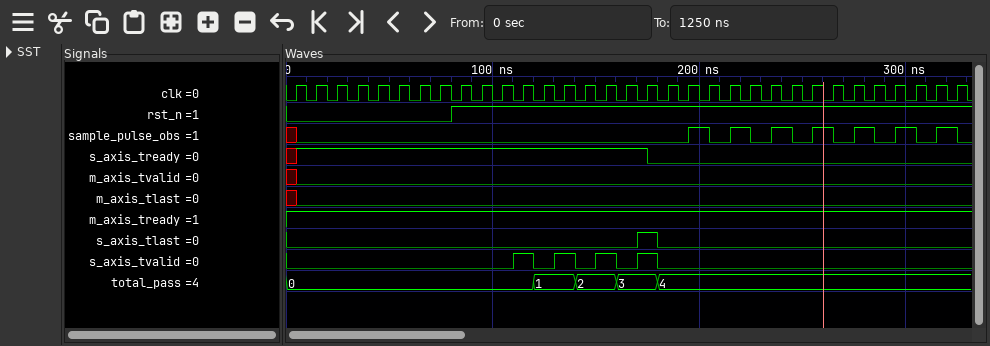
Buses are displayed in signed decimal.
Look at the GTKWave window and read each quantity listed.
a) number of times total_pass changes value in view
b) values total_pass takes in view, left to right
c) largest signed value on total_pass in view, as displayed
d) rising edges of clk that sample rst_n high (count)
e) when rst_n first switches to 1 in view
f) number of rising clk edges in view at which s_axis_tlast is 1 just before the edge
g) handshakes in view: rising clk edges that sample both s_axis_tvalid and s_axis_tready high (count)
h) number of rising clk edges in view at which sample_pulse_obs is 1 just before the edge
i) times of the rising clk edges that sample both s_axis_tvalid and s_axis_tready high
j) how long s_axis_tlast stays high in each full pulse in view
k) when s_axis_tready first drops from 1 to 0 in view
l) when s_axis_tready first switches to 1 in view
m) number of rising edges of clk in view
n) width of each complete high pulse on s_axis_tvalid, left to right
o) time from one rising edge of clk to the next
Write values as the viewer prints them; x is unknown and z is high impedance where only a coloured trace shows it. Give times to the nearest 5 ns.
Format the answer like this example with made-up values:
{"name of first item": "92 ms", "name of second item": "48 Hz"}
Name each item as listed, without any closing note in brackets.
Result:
{"number of times total_pass changes value in view": "4", "values total_pass takes in view, left to right": "0, 1, 2, 3, 4", "largest signed value on total_pass in view, as displayed": "4", "rising edges of clk that sample rst_n high": "25", "when rst_n first switches to 1 in view": "80 ns", "number of rising clk edges in view at which s_axis_tlast is 1 just before the edge": "1", "handshakes in view: rising clk edges that sample both s_axis_tvalid and s_axis_tready high": "4", "number of rising clk edges in view at which sample_pulse_obs is 1 just before the edge": "7", "times of the rising clk edges that sample both s_axis_tvalid and s_axis_tready high": "115 ns, 135 ns, 155 ns, 175 ns", "how long s_axis_tlast stays high in each full pulse in view": "10 ns", "when s_axis_tready first drops from 1 to 0 in view": "175 ns", "when s_axis_tready first switches to 1 in view": "5 ns", "number of rising edges of clk in view": "33", "width of each complete high pulse on s_axis_tvalid, left to right": "10 ns, 10 ns, 10 ns, 10 ns", "time from one rising edge of clk to the next": "10 ns"}
